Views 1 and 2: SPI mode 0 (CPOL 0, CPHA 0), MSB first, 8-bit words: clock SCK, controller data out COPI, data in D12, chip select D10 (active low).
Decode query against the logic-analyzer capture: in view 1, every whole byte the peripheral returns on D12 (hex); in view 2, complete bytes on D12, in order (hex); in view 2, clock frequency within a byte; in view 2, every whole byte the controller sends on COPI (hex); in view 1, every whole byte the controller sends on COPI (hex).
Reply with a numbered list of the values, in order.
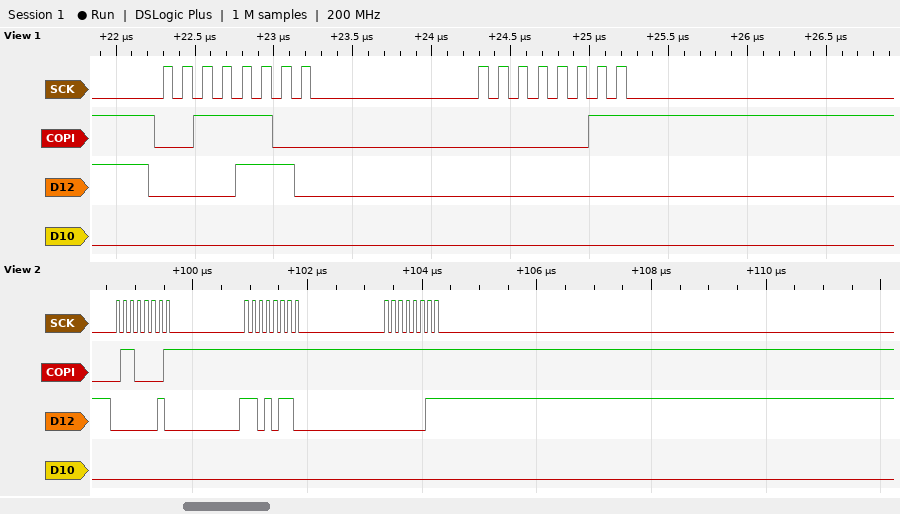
1. 0x0E 0x00
2. 02 D6 03
3. 8 MHz
4. 61 FF FF
5. 0x3C 0x03
